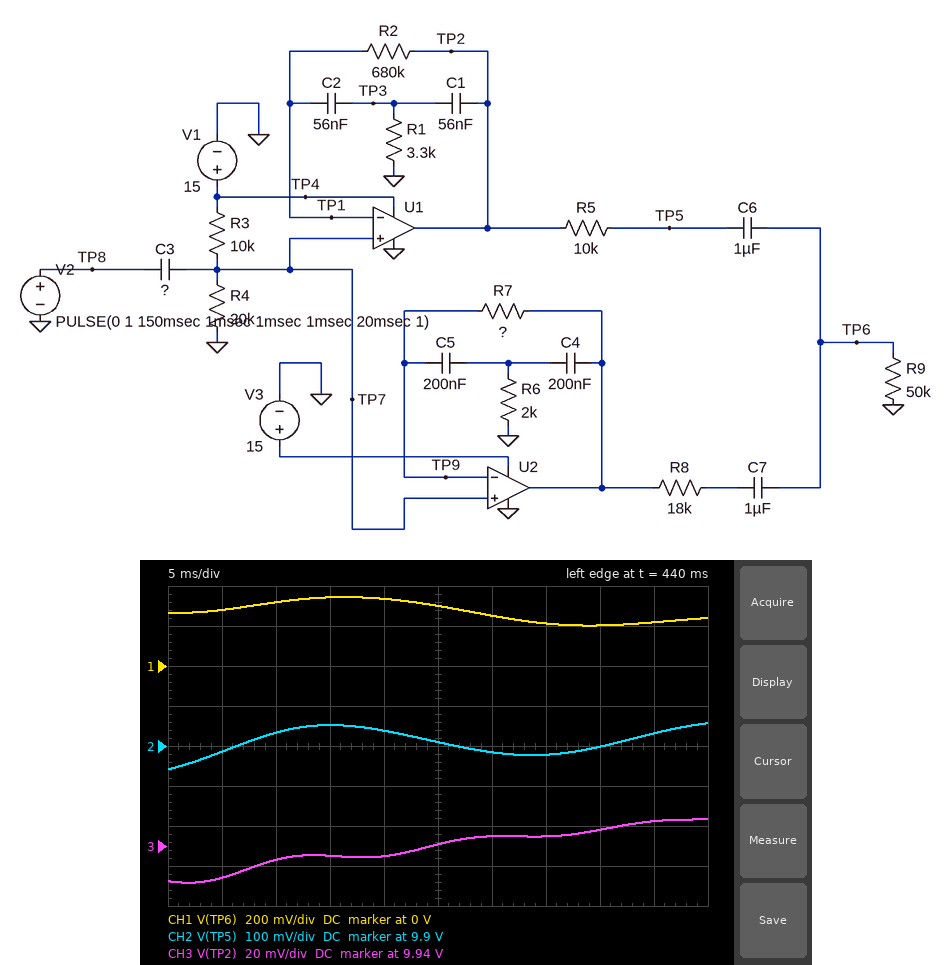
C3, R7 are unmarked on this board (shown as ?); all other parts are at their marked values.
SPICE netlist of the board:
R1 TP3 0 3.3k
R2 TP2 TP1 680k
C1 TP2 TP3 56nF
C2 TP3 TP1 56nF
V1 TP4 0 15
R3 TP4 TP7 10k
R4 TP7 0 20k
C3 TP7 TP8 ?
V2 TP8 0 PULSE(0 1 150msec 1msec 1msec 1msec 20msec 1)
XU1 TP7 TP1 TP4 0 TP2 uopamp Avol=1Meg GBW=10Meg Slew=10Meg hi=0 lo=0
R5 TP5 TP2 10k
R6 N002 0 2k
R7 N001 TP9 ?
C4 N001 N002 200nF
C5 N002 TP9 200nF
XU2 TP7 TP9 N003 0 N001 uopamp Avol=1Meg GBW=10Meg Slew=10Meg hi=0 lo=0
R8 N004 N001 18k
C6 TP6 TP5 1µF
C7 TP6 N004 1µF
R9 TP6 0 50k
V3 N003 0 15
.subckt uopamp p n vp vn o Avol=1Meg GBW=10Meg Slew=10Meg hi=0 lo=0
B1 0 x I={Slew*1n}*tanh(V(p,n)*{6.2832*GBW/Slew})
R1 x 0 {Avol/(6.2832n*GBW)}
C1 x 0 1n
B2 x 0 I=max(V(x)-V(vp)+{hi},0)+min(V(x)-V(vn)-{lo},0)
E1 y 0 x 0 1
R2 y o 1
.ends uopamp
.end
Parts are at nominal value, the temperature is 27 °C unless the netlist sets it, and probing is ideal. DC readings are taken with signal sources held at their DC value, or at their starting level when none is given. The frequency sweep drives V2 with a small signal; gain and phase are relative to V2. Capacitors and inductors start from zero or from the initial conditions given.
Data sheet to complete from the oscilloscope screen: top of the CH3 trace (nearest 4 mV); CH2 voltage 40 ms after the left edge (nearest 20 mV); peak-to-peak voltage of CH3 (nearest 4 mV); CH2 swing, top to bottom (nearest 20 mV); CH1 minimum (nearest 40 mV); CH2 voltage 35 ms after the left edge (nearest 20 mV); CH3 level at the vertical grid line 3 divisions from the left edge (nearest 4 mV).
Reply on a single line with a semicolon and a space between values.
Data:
9.952 V; 9.90 V; 32 mV; 120 mV; 200 mV; 9.88 V; 9.936 V
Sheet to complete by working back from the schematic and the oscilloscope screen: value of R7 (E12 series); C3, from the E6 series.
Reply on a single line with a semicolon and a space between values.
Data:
470 kΩ; 15 µF
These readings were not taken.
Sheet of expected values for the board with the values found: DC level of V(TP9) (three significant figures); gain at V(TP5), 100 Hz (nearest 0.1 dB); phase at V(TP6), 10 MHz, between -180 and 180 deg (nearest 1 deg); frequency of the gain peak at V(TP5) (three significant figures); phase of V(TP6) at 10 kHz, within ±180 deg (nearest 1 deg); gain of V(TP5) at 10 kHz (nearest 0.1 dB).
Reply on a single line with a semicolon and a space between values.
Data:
10.0 V; 19.2 dB; -45 deg; 60.1 Hz; -4 deg; -1.0 dB
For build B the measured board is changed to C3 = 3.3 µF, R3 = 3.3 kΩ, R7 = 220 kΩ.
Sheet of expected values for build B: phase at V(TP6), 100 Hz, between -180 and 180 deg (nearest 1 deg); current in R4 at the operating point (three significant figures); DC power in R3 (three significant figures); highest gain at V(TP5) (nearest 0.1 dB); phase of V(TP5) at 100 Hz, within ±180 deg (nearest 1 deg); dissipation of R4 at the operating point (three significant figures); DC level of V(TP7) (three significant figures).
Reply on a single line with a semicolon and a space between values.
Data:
-66 deg; 644 µA; 1.37 mW; 35.7 dB; -70 deg; 8.29 mW; 12.9 V
